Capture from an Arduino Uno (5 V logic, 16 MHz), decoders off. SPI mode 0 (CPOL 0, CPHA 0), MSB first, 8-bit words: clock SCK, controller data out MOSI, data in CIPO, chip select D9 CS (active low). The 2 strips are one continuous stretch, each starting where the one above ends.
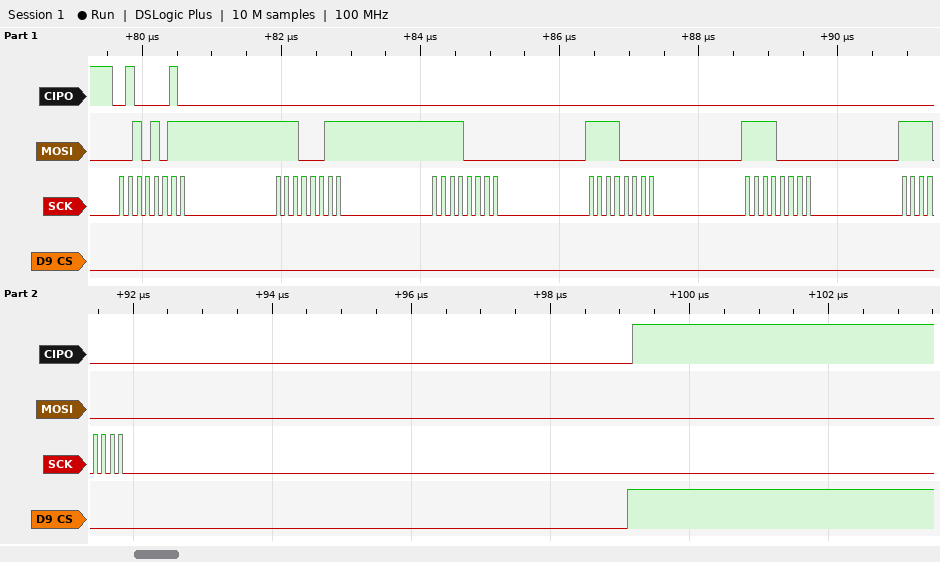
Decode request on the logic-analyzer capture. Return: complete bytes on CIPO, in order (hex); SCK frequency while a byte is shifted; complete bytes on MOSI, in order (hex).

42 00 00 00 00 00
8 MHz
2B E3 F0 F0 F0 F0
